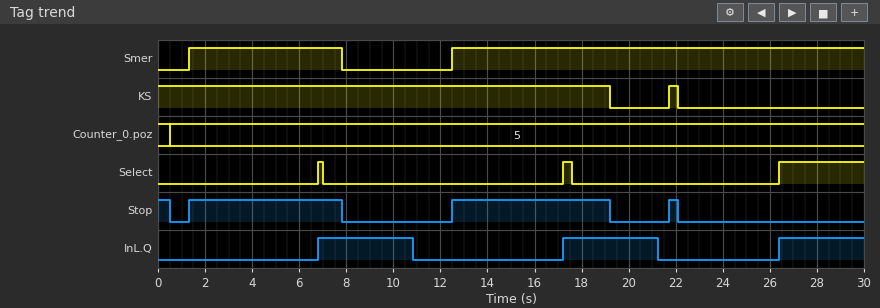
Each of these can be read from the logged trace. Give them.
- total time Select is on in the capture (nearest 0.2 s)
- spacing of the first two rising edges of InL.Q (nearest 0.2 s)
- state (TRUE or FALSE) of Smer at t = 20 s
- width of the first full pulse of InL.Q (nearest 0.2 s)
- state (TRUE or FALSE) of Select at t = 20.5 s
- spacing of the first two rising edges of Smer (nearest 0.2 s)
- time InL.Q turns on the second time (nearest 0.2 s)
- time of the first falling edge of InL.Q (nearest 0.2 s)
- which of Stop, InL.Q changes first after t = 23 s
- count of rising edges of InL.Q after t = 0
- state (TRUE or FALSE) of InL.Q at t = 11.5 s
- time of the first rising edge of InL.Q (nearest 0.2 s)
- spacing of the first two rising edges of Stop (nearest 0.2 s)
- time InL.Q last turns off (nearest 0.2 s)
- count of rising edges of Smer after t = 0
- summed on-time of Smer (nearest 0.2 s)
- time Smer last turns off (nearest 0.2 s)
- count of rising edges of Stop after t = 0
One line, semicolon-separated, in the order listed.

4.2 s; 10.4 s; TRUE; 4.0 s; FALSE; 11.2 s; 17.2 s; 10.8 s; InL.Q; 3; FALSE; 6.8 s; 11.2 s; 21.2 s; 2; 24.0 s; 7.8 s; 3
